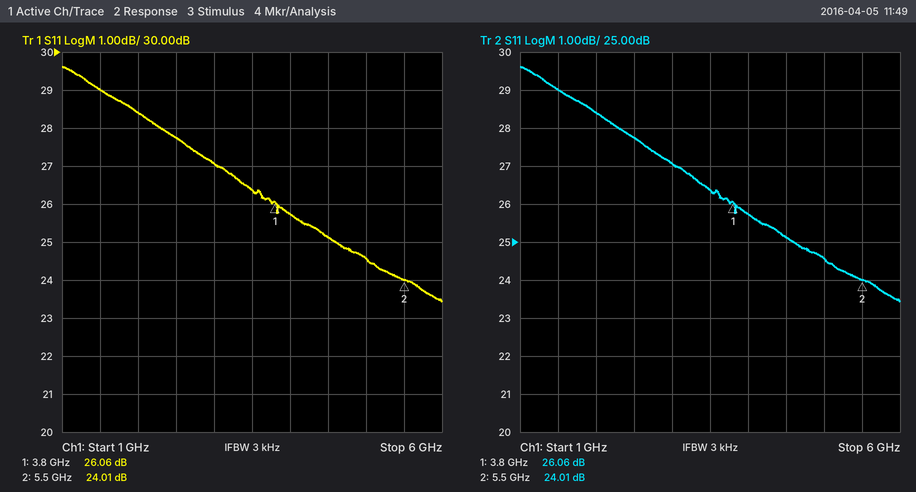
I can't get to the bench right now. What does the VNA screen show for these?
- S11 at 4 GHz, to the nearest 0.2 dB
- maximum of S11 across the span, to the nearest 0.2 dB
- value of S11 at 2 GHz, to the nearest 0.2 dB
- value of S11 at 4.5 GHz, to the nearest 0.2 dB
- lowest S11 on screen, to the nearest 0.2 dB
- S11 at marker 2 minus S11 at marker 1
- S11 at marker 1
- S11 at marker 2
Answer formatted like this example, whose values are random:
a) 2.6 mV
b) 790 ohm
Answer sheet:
a) 25.8 dB
b) 29.6 dB
c) 28.4 dB
d) 25.2 dB
e) 23.4 dB
f) -2.05 dB
g) 26.06 dB
h) 24.01 dB
